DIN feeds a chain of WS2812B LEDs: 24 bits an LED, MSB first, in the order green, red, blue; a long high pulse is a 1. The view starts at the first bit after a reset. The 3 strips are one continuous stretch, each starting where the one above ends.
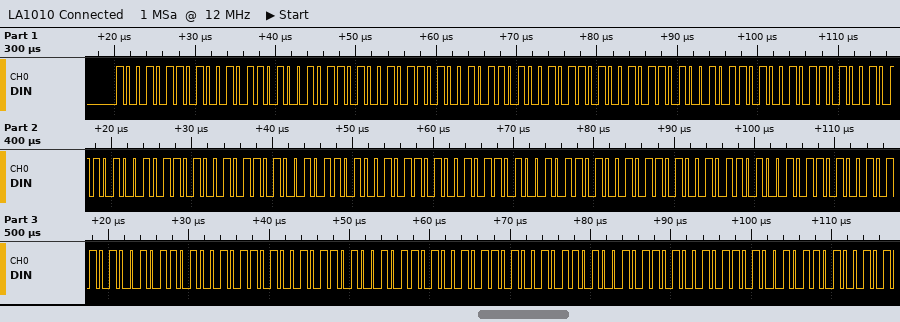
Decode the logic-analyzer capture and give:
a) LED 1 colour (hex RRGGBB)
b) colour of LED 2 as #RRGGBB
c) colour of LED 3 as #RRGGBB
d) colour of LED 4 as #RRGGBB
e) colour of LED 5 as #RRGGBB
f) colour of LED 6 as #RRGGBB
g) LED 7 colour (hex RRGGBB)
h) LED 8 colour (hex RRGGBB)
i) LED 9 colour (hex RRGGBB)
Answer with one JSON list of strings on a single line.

["#969696", "#969696", "#969696", "#969696", "#969696", "#969696", "#969696", "#969696", "#969696"]
